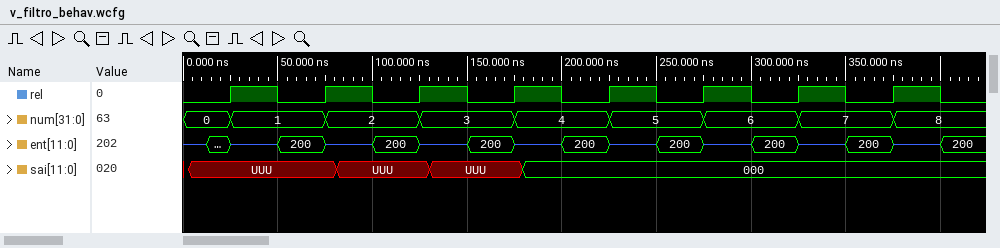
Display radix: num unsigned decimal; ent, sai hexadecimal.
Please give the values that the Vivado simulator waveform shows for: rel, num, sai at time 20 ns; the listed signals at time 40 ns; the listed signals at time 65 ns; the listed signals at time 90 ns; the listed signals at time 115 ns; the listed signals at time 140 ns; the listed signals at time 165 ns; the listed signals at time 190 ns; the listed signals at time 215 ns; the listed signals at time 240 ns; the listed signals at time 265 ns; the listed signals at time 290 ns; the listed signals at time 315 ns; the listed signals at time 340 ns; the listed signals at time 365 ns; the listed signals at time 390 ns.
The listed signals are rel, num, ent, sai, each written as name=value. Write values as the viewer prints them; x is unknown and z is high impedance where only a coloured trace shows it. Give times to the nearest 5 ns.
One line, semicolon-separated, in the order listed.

rel=0, num=0, sai=UUU; rel=1, num=1, ent=z, sai=UUU; rel=0, num=1, ent=200, sai=UUU; rel=1, num=2, ent=z, sai=UUU; rel=0, num=2, ent=200, sai=UUU; rel=1, num=3, ent=z, sai=UUU; rel=0, num=3, ent=200, sai=UUU; rel=1, num=4, ent=z, sai=000; rel=0, num=4, ent=200, sai=000; rel=1, num=5, ent=z, sai=000; rel=0, num=5, ent=200, sai=000; rel=1, num=6, ent=z, sai=000; rel=0, num=6, ent=200, sai=000; rel=1, num=7, ent=z, sai=000; rel=0, num=7, ent=200, sai=000; rel=1, num=8, ent=z, sai=000
